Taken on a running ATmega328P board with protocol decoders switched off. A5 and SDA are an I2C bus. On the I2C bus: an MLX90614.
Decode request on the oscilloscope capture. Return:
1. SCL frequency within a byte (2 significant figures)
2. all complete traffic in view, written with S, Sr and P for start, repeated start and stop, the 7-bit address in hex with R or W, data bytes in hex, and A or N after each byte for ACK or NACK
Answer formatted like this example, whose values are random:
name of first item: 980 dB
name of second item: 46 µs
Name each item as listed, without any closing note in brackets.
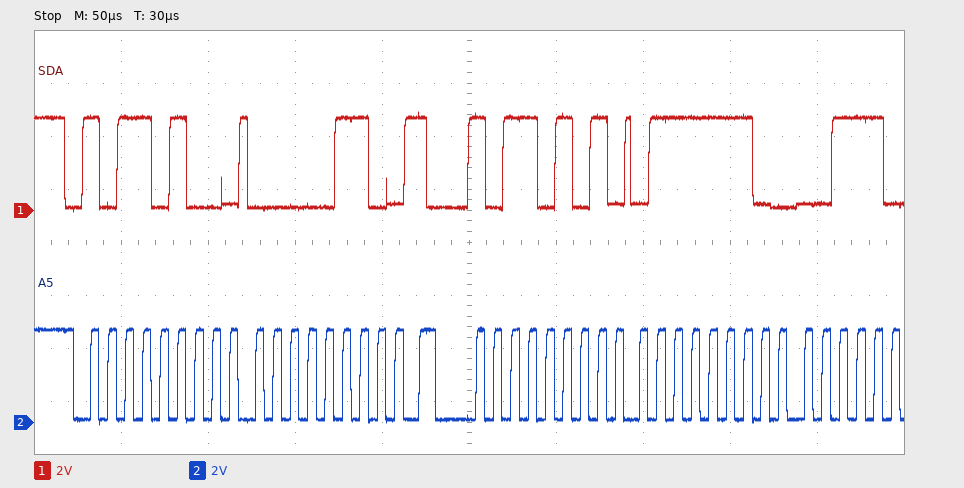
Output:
SCL frequency within a byte: 100 kHz
all complete traffic in view, written with S, Sr and P for start, repeated start and stop, the 7-bit address in hex with R or W, data bytes in hex, and A or N after each byte for ACK or NACK: S 5AW A 06 A Sr 5AR A 7E A
